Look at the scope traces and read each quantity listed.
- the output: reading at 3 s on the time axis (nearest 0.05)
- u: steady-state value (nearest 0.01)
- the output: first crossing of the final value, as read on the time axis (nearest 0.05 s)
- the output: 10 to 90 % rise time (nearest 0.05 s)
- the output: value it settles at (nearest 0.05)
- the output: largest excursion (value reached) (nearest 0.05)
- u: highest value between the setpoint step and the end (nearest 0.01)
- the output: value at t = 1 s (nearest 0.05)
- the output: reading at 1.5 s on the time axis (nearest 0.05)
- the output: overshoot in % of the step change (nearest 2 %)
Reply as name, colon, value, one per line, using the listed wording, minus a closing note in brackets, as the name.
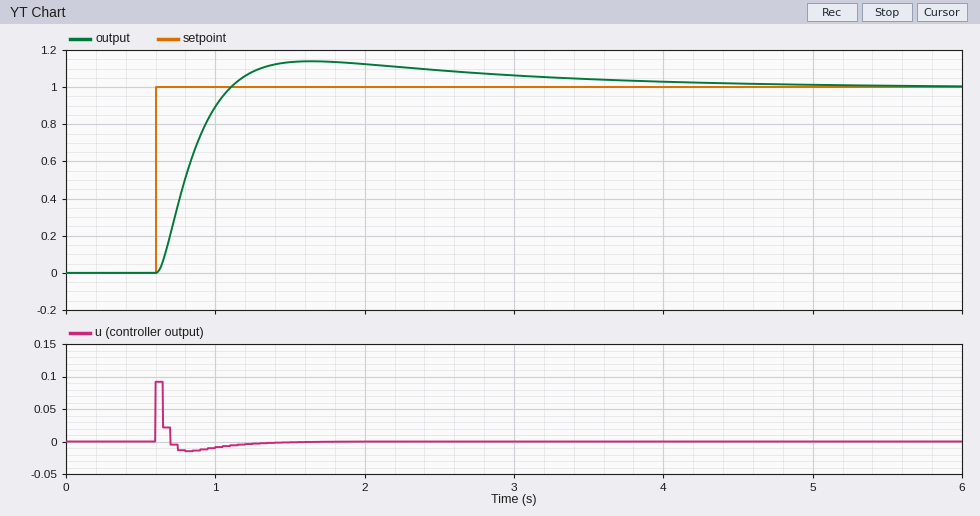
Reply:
the output: reading at 3 s on the time axis: 1.05
u: steady-state value: 0.00
the output: first crossing of the final value, as read on the time axis: 1.10 s
the output: 10 to 90 % rise time: 0.35 s
the output: value it settles at: 1.00
the output: largest excursion (value reached): 1.15
u: highest value between the setpoint step and the end: 0.09
the output: value at t = 1 s: 0.90
the output: reading at 1.5 s on the time axis: 1.15
the output: overshoot in % of the step change: 14 %
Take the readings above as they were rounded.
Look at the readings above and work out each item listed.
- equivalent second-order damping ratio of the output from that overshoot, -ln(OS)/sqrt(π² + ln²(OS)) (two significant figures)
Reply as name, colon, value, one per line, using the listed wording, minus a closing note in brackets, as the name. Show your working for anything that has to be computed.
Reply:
equivalent second-order damping ratio of the output from that overshoot, -ln(OS)/sqrt(π² + ln²(OS)): ln(0.14) = -1.966; 1.966 / sqrt(9.870 + 3.866) = 0.53
